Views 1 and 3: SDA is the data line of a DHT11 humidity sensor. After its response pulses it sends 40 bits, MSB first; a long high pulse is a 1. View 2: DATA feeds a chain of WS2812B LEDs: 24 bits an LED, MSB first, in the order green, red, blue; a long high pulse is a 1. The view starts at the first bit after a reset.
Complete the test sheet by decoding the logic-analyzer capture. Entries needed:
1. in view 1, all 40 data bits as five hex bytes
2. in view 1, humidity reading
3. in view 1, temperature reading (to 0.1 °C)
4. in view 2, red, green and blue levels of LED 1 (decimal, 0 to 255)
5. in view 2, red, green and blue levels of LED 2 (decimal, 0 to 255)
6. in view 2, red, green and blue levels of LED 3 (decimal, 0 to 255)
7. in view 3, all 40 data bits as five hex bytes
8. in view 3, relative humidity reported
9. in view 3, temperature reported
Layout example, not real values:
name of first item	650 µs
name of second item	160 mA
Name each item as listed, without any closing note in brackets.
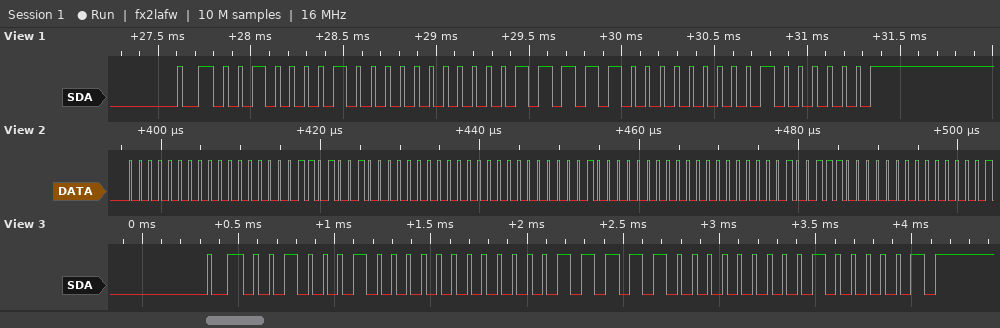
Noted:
in view 1, all 40 data bits as five hex bytes	21 00 1F 00 40
in view 1, humidity reading	33 %
in view 1, temperature reading	31.0 °C
in view 2, red, green and blue levels of LED 1	0, 0, 105
in view 2, red, green and blue levels of LED 2	0, 0, 2
in view 2, red, green and blue levels of LED 3	0, 0, 39
in view 3, all 40 data bits as five hex bytes	22 00 1F 00 41
in view 3, relative humidity reported	34 %
in view 3, temperature reported	31.0 °C
